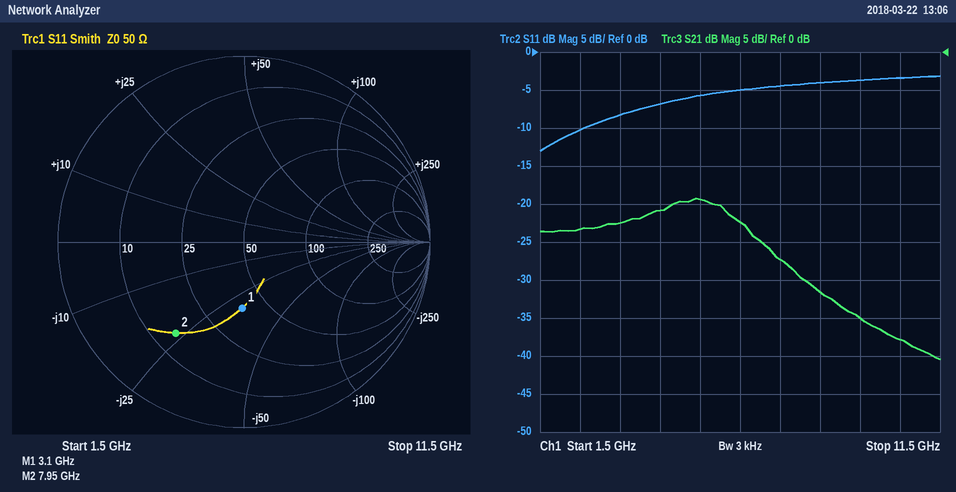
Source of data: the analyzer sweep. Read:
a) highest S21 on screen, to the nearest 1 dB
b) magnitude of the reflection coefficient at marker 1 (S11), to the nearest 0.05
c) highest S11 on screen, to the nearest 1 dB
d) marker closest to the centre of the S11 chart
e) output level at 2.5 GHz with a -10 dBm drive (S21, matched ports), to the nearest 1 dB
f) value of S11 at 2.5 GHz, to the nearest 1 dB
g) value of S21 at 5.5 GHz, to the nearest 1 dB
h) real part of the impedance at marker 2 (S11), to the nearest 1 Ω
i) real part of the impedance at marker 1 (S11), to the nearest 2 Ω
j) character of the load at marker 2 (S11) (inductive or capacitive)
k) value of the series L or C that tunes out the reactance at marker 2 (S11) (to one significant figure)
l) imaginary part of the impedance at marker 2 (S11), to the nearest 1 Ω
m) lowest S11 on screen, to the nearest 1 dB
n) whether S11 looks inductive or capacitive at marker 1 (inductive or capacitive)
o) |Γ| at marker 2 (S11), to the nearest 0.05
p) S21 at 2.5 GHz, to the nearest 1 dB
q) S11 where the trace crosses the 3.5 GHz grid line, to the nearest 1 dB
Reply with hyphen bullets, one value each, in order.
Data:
- -19 dB
- 0.35
- -3 dB
- marker 1
- -33 dBm
- -10 dB
- -19 dB
- 15 Ω
- 38 Ω
- capacitive
- 500 pH
- -23 Ω
- -13 dB
- capacitive
- 0.60
- -23 dB
- -8 dB
